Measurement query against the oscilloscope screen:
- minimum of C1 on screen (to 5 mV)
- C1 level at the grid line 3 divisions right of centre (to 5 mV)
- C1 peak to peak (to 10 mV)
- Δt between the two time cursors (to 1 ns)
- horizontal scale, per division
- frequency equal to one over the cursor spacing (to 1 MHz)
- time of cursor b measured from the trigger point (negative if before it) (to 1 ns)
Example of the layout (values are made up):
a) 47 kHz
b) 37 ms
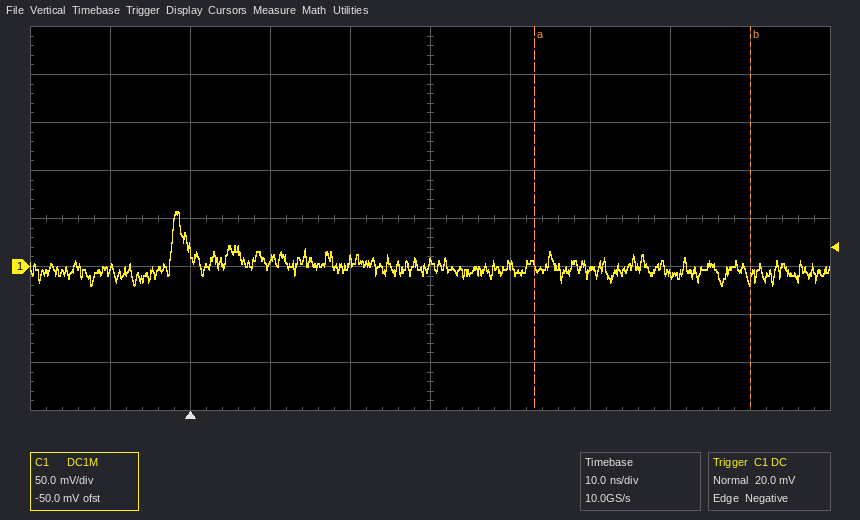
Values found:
a) -20 mV
b) -10 mV
c) 80 mV
d) 27 ns
e) 10 ns
f) 37 MHz
g) +70 ns
